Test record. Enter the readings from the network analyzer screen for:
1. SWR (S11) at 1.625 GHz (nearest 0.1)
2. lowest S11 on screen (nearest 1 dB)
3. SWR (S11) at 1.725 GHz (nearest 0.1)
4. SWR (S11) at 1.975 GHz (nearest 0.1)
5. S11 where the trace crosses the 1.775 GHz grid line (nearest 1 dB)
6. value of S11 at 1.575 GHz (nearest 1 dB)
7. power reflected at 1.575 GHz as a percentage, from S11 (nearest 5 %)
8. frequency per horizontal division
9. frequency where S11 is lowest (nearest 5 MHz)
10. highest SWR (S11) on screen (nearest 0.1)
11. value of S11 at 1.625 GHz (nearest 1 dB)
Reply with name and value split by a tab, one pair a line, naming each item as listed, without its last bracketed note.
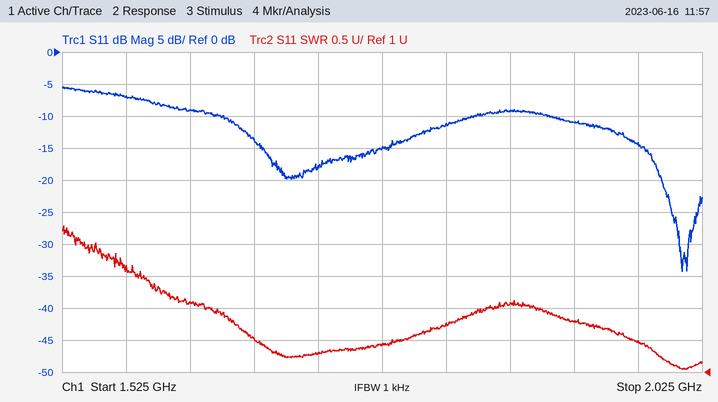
SWR (S11) at 1.625 GHz	2.1
lowest S11 on screen	-34 dB
SWR (S11) at 1.725 GHz	1.3
SWR (S11) at 1.975 GHz	1.5
S11 where the trace crosses the 1.775 GHz grid line	-15 dB
value of S11 at 1.575 GHz	-7 dB
power reflected at 1.575 GHz as a percentage, from S11	20 %
frequency per horizontal division	50 MHz
frequency where S11 is lowest	2.010 GHz
highest SWR (S11) on screen	3.3
value of S11 at 1.625 GHz	-9 dB
